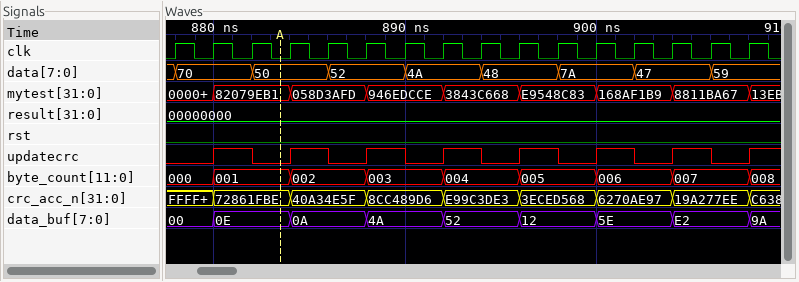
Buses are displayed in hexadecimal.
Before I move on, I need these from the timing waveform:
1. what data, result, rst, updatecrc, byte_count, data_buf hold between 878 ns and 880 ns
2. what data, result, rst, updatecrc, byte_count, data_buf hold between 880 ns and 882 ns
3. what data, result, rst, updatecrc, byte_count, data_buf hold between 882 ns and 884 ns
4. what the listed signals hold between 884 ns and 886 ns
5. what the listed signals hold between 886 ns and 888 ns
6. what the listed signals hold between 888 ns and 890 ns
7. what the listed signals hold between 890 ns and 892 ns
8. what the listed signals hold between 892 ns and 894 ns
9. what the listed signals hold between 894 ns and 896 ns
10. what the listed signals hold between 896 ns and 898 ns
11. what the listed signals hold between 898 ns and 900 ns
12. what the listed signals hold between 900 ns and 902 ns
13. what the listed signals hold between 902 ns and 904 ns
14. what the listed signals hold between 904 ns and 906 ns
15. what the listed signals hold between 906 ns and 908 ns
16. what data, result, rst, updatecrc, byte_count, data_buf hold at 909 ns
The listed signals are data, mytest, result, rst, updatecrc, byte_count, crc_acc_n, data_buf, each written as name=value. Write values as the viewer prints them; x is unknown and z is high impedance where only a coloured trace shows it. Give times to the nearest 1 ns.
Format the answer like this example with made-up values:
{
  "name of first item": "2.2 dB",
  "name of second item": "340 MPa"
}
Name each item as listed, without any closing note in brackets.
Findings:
{
  "what data, result, rst, updatecrc, byte_count, data_buf hold between 878 ns and 880 ns": "data=70, result=00000000, rst=0, updatecrc=0, byte_count=000, data_buf=00",
  "what data, result, rst, updatecrc, byte_count, data_buf hold between 880 ns and 882 ns": "data=70, result=00000000, rst=0, updatecrc=1, byte_count=001, data_buf=0E",
  "what data, result, rst, updatecrc, byte_count, data_buf hold between 882 ns and 884 ns": "data=50, result=00000000, rst=0, updatecrc=0, byte_count=001, data_buf=0E",
  "what the listed signals hold between 884 ns and 886 ns": "data=50, mytest=058D3AFD, result=00000000, rst=0, updatecrc=1, byte_count=002, crc_acc_n=40A34E5F, data_buf=0A",
  "what the listed signals hold between 886 ns and 888 ns": "data=52, mytest=058D3AFD, result=00000000, rst=0, updatecrc=0, byte_count=002, crc_acc_n=40A34E5F, data_buf=0A",
  "what the listed signals hold between 888 ns and 890 ns": "data=52, mytest=946EDCCE, result=00000000, rst=0, updatecrc=1, byte_count=003, crc_acc_n=8CC489D6, data_buf=4A",
  "what the listed signals hold between 890 ns and 892 ns": "data=4A, mytest=946EDCCE, result=00000000, rst=0, updatecrc=0, byte_count=003, crc_acc_n=8CC489D6, data_buf=4A",
  "what the listed signals hold between 892 ns and 894 ns": "data=4A, mytest=3843C668, result=00000000, rst=0, updatecrc=1, byte_count=004, crc_acc_n=E99C3DE3, data_buf=52",
  "what the listed signals hold between 894 ns and 896 ns": "data=48, mytest=3843C668, result=00000000, rst=0, updatecrc=0, byte_count=004, crc_acc_n=E99C3DE3, data_buf=52",
  "what the listed signals hold between 896 ns and 898 ns": "data=48, mytest=E9548C83, result=00000000, rst=0, updatecrc=1, byte_count=005, crc_acc_n=3ECED568, data_buf=12",
  "what the listed signals hold between 898 ns and 900 ns": "data=7A, mytest=E9548C83, result=00000000, rst=0, updatecrc=0, byte_count=005, crc_acc_n=3ECED568, data_buf=12",
  "what the listed signals hold between 900 ns and 902 ns": "data=7A, mytest=168AF1B9, result=00000000, rst=0, updatecrc=1, byte_count=006, crc_acc_n=6270AE97, data_buf=5E",
  "what the listed signals hold between 902 ns and 904 ns": "data=47, mytest=168AF1B9, result=00000000, rst=0, updatecrc=0, byte_count=006, crc_acc_n=6270AE97, data_buf=5E",
  "what the listed signals hold between 904 ns and 906 ns": "data=47, mytest=8811BA67, result=00000000, rst=0, updatecrc=1, byte_count=007, crc_acc_n=19A277EE, data_buf=E2",
  "what the listed signals hold between 906 ns and 908 ns": "data=59, mytest=8811BA67, result=00000000, rst=0, updatecrc=0, byte_count=007, crc_acc_n=19A277EE, data_buf=E2",
  "what data, result, rst, updatecrc, byte_count, data_buf hold at 909 ns": "data=59, result=00000000, rst=0, updatecrc=1, byte_count=008, data_buf=9A"
}
